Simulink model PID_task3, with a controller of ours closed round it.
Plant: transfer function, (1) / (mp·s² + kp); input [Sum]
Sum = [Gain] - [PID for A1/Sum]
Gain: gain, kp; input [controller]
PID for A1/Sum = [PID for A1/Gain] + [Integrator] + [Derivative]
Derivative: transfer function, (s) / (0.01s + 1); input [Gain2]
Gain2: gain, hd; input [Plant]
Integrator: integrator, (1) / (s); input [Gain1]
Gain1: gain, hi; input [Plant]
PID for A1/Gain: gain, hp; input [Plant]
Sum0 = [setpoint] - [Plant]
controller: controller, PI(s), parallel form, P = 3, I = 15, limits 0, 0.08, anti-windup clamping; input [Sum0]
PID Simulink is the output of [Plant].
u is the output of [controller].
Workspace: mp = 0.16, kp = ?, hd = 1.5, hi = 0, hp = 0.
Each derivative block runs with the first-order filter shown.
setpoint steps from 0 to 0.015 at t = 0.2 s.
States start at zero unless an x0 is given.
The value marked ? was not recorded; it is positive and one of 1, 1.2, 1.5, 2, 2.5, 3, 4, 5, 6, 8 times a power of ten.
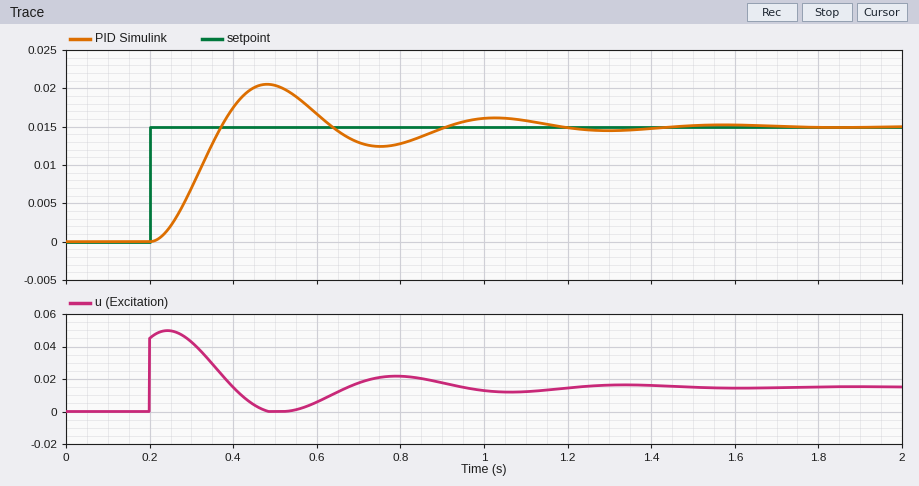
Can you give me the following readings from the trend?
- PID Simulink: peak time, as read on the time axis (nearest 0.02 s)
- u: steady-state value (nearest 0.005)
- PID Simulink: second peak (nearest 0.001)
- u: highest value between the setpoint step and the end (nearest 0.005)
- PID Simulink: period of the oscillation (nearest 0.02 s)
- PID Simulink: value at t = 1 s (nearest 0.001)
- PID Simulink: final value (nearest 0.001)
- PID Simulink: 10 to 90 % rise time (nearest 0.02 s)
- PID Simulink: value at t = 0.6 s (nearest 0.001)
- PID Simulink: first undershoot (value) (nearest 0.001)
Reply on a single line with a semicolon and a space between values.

0.48 s; 0.015; 0.016; 0.050; 0.54 s; 0.016; 0.015; 0.12 s; 0.017; 0.012
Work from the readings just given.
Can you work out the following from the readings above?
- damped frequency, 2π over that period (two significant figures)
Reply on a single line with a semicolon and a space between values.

12 rad/s
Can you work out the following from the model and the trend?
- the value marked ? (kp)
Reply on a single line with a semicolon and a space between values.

6
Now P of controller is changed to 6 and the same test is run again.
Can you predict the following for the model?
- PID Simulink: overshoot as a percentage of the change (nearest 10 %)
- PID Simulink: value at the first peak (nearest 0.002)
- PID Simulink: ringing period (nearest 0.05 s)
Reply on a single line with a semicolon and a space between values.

30 %; 0.020; 0.45 s
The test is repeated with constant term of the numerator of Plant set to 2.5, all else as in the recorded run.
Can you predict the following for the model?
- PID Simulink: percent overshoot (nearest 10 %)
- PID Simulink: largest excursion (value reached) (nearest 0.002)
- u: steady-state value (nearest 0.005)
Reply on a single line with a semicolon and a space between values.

20 %; 0.018; 0.005
